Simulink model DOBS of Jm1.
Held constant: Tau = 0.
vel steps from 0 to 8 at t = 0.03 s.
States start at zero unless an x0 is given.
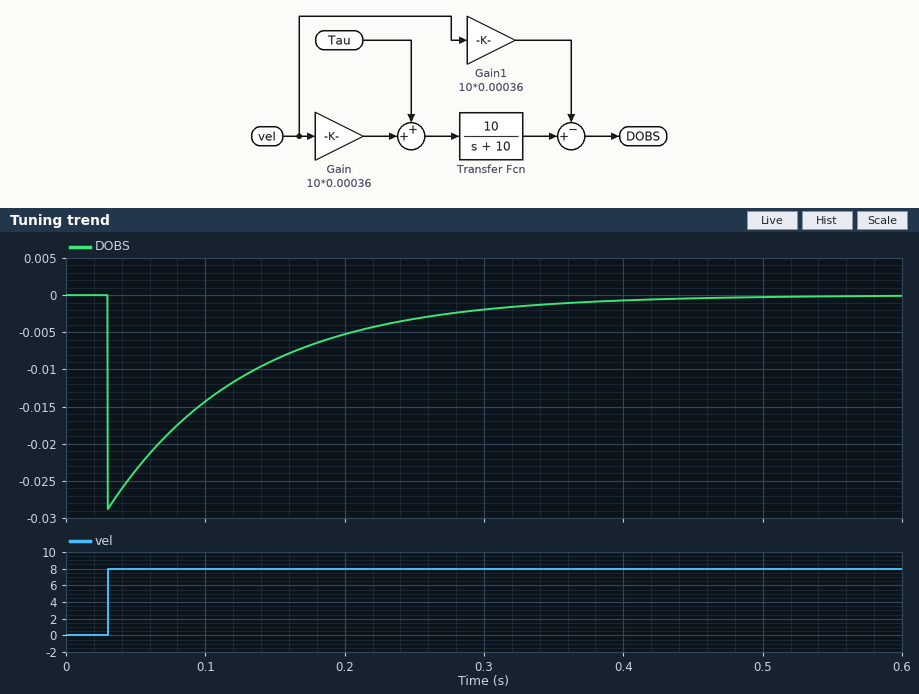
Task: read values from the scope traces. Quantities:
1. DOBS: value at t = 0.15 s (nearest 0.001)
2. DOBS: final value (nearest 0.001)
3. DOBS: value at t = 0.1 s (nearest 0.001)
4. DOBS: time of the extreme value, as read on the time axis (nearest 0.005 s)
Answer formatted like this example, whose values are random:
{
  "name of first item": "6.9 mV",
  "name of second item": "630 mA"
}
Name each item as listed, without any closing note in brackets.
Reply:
{
  "DOBS: value at t = 0.15 s": "-0.009",
  "DOBS: final value": "0.000",
  "DOBS: value at t = 0.1 s": "-0.014",
  "DOBS: time of the extreme value, as read on the time axis": "0.030 s"
}
